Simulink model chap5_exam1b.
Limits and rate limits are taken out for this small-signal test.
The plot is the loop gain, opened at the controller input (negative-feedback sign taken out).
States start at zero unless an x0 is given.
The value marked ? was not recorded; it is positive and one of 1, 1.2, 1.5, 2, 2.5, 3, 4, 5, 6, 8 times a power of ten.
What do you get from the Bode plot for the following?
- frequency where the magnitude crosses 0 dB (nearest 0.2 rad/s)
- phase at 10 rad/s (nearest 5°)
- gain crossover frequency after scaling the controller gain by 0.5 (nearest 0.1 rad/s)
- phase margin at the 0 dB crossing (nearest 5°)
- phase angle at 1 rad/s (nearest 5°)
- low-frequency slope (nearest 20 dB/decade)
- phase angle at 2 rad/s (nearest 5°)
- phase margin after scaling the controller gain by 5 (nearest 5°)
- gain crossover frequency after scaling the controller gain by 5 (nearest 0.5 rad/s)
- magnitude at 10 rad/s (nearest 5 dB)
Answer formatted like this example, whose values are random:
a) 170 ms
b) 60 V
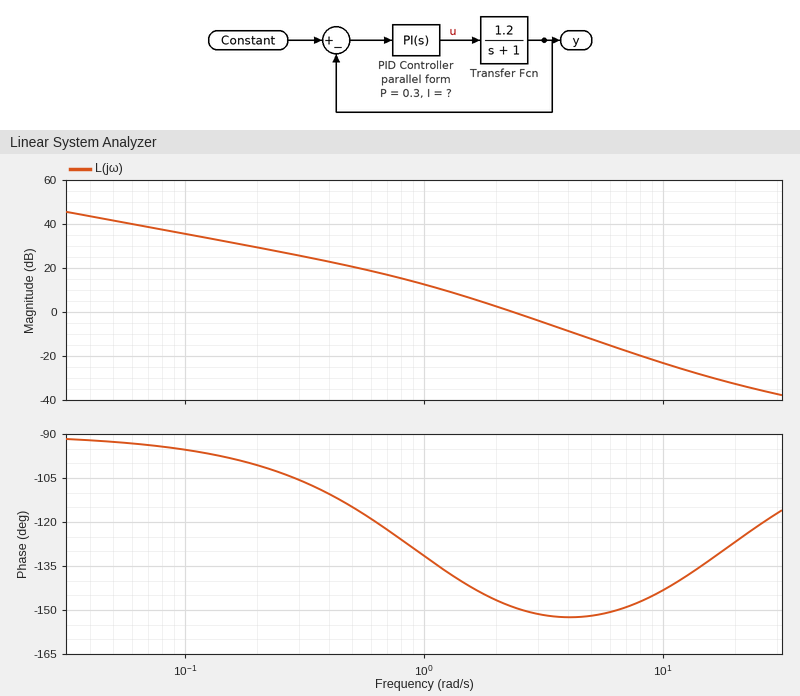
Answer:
a) 2.4 rad/s
b) -145°
c) 1.6 rad/s
d) 30°
e) -130°
f) -20 dB/decade
g) -145°
h) 30°
i) 5.5 rad/s
j) -25 dB
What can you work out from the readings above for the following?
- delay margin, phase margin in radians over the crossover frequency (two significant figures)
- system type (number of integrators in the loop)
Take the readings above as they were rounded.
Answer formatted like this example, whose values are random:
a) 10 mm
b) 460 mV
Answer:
a) 0.22 s
b) 1
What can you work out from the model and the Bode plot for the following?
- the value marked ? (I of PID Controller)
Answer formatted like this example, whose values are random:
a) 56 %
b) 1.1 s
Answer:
a) 5
